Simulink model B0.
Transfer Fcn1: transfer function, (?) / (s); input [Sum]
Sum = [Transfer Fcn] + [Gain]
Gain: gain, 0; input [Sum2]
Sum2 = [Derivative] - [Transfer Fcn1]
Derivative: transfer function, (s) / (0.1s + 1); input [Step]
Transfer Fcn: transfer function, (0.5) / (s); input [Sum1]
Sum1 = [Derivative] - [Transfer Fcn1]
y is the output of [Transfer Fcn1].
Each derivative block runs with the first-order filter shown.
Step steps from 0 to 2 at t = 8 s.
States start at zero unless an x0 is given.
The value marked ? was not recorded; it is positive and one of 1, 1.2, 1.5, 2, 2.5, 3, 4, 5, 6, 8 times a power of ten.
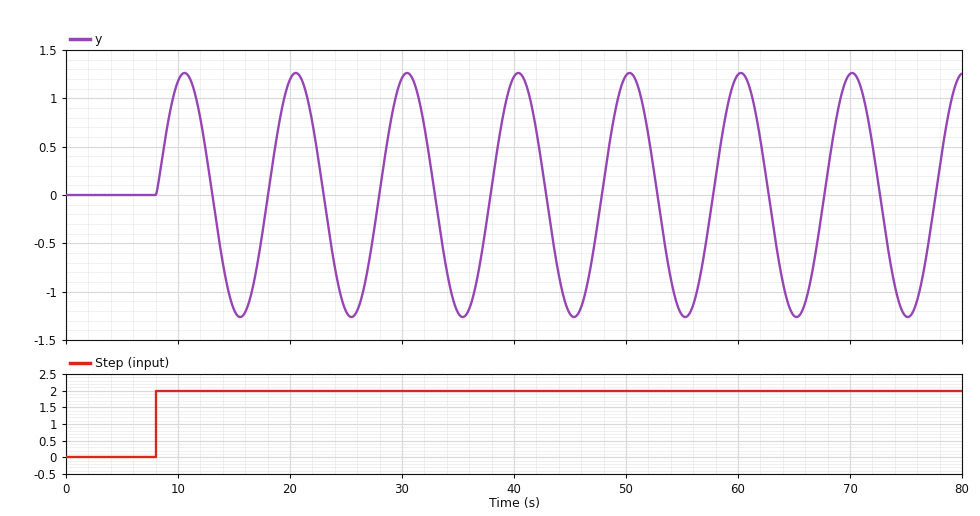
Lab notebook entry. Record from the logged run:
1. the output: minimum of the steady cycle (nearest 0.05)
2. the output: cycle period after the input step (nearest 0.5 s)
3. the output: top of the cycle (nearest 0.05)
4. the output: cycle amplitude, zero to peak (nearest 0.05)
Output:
-1.25
10.0 s
1.25
1.25
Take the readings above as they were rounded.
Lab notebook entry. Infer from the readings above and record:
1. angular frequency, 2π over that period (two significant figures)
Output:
0.63 rad/s
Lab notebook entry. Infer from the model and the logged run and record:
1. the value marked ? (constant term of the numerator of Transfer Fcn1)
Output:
0.8
